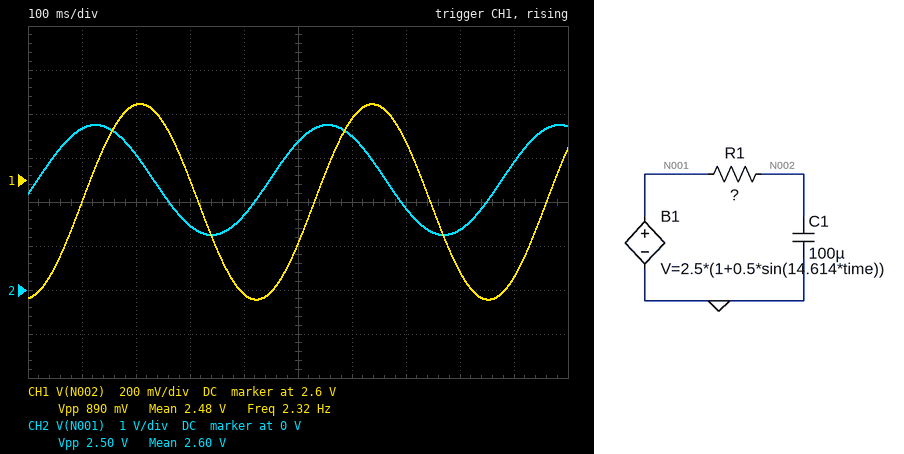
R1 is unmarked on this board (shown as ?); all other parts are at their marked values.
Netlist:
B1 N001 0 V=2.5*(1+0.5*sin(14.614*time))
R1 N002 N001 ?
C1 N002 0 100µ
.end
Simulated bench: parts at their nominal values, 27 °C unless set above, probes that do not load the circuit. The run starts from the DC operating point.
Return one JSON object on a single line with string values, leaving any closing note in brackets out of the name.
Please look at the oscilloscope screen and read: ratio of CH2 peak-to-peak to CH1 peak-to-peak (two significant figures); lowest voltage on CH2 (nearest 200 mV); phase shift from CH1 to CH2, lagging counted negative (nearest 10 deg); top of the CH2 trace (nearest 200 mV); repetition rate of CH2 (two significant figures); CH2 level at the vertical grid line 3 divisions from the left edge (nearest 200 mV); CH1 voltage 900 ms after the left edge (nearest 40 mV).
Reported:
{"ratio of CH2 peak-to-peak to CH1 peak-to-peak": "2.8", "lowest voltage on CH2": "1.2 V", "phase shift from CH1 to CH2, lagging counted negative": "70 deg", "top of the CH2 trace": "3.8 V", "repetition rate of CH2": "2.3 Hz", "CH2 level at the vertical grid line 3 divisions from the left edge": "1.4 V", "CH1 voltage 900 ms after the left edge": "2.16 V"}
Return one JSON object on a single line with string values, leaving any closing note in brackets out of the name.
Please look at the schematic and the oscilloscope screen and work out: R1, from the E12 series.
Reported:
{"R1, from the E12 series": "1.8 kΩ"}
